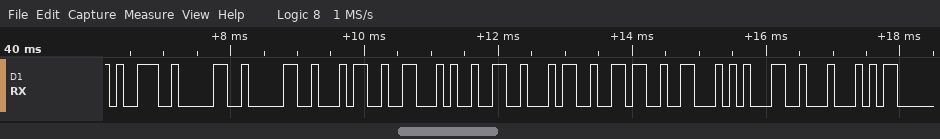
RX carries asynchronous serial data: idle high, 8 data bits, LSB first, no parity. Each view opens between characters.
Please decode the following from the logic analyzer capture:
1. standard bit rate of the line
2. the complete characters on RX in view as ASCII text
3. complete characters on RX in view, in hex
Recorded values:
9600 baud
"9004F246F1D"
39, 30, 30, 34, 46, 32, 34, 36, 46, 31, 44
